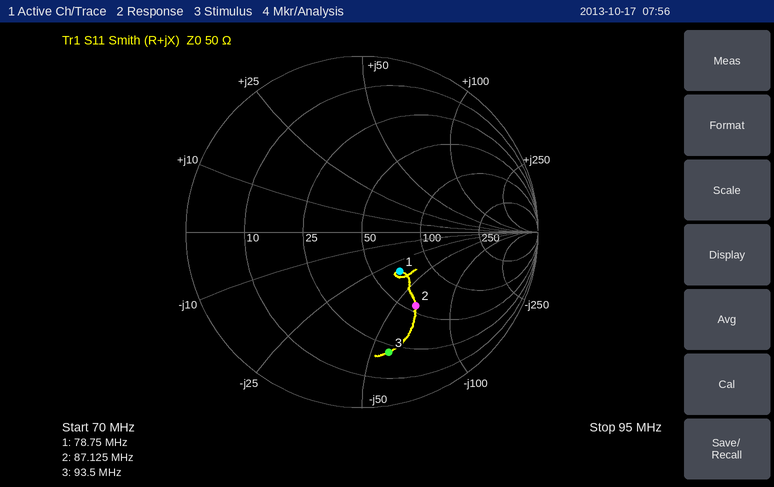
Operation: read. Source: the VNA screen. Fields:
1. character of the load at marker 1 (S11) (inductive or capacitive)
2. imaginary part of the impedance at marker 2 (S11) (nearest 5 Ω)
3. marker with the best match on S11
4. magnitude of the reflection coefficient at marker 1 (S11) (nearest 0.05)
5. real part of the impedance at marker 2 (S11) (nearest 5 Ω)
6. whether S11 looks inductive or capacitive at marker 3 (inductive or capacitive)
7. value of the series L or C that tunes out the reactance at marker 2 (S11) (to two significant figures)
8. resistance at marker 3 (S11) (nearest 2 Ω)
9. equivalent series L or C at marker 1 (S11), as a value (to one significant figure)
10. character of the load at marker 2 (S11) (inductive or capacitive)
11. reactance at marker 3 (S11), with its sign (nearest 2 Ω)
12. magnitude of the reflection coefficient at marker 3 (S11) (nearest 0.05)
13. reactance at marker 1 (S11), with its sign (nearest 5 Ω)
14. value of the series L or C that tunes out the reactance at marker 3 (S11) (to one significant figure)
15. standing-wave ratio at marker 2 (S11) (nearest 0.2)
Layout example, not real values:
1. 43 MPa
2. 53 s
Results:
1. capacitive
2. -65 Ω
3. marker 1
4. 0.30
5. 55 Ω
6. capacitive
7. 120 nH
8. 22 Ω
9. 60 pF
10. capacitive
11. -58 Ω
12. 0.70
13. -35 Ω
14. 100 nH
15. 3.2
